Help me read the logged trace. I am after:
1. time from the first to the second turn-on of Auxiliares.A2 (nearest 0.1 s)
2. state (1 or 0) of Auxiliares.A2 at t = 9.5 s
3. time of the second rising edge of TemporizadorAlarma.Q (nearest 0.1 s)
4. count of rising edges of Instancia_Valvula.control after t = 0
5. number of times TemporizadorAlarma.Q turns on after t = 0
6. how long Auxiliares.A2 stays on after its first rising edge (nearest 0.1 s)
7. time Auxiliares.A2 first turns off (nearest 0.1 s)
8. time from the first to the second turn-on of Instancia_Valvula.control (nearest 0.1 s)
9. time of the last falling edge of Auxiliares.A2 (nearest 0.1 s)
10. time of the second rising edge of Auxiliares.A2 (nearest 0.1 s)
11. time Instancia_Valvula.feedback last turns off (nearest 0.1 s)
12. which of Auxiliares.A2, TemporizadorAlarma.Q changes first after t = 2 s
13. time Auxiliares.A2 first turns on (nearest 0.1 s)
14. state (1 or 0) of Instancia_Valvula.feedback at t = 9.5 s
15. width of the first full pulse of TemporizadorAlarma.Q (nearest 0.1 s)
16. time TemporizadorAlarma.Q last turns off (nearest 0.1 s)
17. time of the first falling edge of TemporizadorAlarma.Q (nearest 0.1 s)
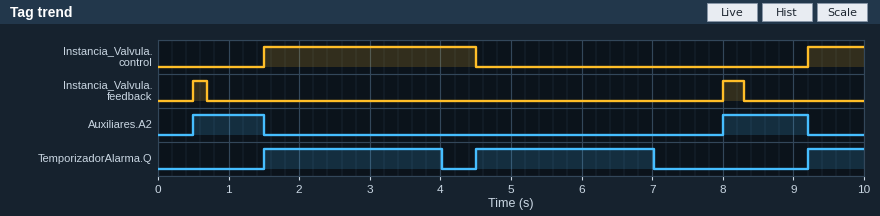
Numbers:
7.5 s
0
4.5 s
2
3
1.0 s
1.5 s
7.7 s
9.2 s
8.0 s
8.3 s
TemporizadorAlarma.Q
0.5 s
0
2.5 s
7.0 s
4.0 s
